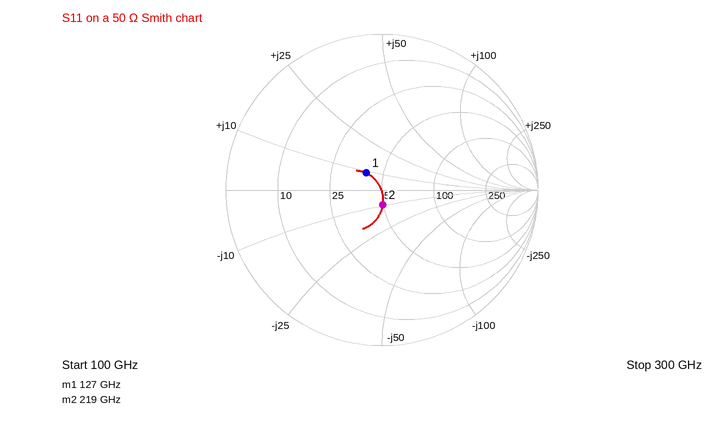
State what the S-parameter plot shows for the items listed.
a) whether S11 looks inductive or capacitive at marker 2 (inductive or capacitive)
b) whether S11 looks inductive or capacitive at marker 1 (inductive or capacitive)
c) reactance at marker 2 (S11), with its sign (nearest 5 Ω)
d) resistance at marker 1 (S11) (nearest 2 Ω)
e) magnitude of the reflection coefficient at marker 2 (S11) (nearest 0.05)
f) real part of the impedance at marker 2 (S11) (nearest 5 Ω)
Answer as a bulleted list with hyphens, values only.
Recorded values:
- capacitive
- inductive
- -10 Ω
- 40 Ω
- 0.10
- 50 Ω
